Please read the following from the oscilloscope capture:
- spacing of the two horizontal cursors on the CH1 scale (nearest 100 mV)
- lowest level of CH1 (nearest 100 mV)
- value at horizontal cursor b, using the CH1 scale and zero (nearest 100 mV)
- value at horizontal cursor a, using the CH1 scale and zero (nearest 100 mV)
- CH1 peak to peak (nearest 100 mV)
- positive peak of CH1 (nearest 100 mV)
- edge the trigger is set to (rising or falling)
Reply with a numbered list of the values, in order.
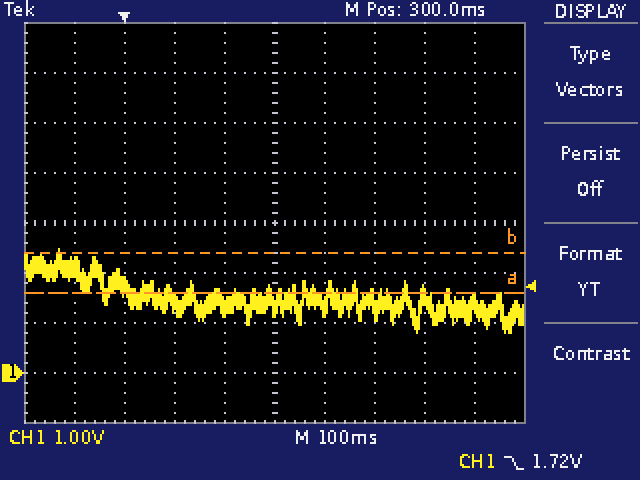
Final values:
1. 800 mV
2. 800 mV
3. 2.4 V
4. 1.6 V
5. 1.7 V
6. 2.5 V
7. falling
